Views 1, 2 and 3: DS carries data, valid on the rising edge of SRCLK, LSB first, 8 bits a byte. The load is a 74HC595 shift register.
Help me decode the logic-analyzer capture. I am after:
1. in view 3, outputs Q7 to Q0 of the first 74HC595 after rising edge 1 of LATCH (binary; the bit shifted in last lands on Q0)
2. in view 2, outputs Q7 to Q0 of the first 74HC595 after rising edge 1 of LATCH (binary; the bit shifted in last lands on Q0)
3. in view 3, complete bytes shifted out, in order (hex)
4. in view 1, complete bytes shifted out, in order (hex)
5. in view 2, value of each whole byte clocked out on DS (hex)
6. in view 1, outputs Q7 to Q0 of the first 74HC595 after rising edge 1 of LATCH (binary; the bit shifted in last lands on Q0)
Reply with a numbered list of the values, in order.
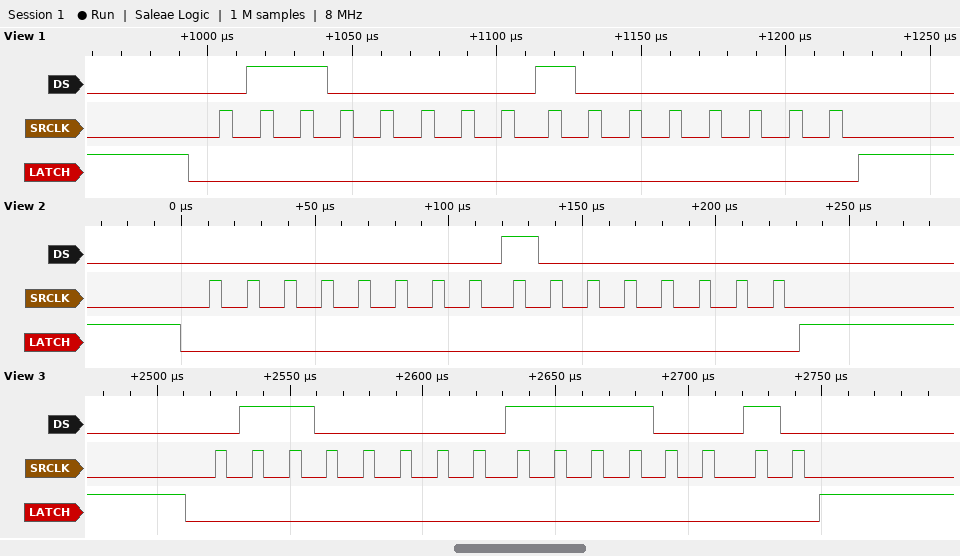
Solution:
1. 11110010
2. 10000000
3. 06 4F
4. 0x06 0x01
5. 0x00 0x01
6. 10000000
